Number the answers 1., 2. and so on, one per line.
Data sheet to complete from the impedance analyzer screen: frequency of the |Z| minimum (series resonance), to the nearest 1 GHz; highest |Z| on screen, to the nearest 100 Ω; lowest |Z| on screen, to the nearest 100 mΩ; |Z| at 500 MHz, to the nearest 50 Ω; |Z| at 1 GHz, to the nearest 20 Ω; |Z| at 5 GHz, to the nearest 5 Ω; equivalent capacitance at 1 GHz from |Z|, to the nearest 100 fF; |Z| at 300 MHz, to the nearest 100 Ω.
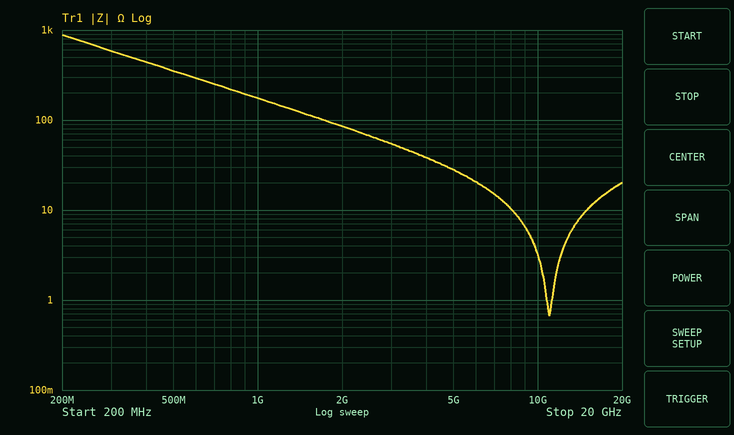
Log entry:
1. 11 GHz
2. 900 Ω
3. 700 mΩ
4. 350 Ω
5. 180 Ω
6. 30 Ω
7. 900 fF
8. 600 Ω
